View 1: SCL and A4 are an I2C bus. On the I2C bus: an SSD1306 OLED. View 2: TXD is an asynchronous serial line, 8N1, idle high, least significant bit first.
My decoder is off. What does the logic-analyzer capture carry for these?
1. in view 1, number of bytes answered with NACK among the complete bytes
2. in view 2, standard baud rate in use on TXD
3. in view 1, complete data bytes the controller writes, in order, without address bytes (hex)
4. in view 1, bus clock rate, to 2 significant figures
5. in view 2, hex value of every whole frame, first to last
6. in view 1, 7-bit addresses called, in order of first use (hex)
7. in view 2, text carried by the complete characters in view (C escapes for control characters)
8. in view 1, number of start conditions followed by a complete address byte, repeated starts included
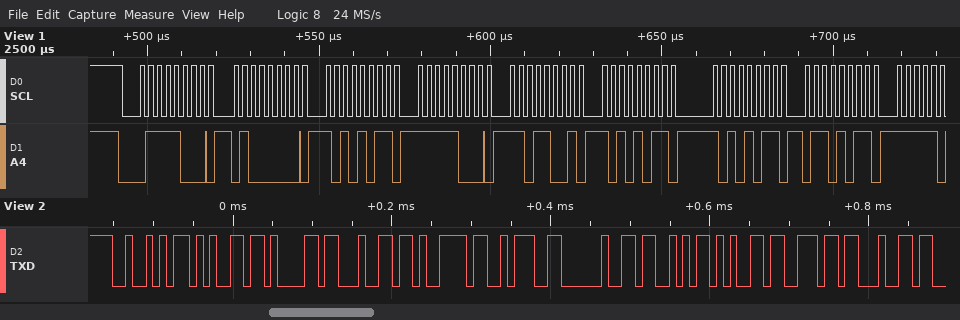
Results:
0
115200 baud
40 AB F8 D9 AB AB 6B
400 kHz
52 65 61 64 79 3A 20 53 65 6E 64
0x3C
"Ready: Send"
1
